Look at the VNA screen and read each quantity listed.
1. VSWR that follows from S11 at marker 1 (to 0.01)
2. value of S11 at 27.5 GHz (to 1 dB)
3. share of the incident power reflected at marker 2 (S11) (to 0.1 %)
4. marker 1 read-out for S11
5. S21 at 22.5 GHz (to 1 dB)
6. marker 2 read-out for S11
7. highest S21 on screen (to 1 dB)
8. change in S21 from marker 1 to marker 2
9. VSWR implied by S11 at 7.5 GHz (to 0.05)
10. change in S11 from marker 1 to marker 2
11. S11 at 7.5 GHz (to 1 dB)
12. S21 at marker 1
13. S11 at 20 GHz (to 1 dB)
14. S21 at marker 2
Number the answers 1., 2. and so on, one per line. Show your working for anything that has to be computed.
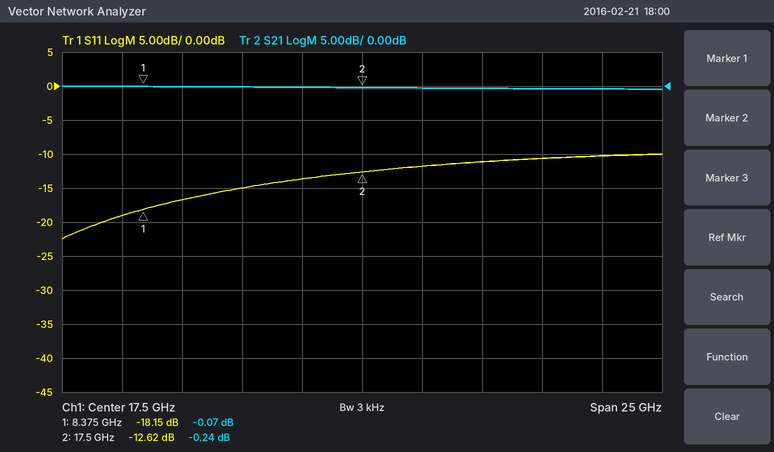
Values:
1. (1 + 0.1237)/(1 − 0.1237) ≈ 1.28
2. -10 dB
3. 10^(-12.62/10) ≈ 5.5 %
4. -18.15 dB
5. 0 dB
6. -12.62 dB
7. 0 dB
8. -0.24 − (-0.07) = -0.17 dB
9. |Γ| = 10^(-19/20) = 0.1122; VSWR = (1 + 0.1122)/(1 − 0.1122) ≈ 1.25
10. -12.62 − (-18.15) = 5.53 dB
11. -19 dB
12. -0.07 dB
13. -12 dB
14. -0.24 dB
